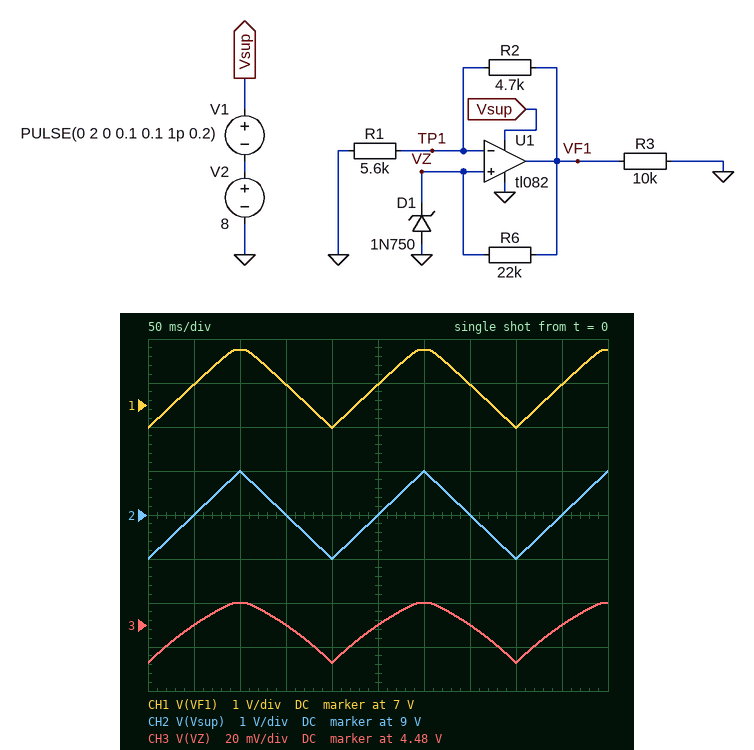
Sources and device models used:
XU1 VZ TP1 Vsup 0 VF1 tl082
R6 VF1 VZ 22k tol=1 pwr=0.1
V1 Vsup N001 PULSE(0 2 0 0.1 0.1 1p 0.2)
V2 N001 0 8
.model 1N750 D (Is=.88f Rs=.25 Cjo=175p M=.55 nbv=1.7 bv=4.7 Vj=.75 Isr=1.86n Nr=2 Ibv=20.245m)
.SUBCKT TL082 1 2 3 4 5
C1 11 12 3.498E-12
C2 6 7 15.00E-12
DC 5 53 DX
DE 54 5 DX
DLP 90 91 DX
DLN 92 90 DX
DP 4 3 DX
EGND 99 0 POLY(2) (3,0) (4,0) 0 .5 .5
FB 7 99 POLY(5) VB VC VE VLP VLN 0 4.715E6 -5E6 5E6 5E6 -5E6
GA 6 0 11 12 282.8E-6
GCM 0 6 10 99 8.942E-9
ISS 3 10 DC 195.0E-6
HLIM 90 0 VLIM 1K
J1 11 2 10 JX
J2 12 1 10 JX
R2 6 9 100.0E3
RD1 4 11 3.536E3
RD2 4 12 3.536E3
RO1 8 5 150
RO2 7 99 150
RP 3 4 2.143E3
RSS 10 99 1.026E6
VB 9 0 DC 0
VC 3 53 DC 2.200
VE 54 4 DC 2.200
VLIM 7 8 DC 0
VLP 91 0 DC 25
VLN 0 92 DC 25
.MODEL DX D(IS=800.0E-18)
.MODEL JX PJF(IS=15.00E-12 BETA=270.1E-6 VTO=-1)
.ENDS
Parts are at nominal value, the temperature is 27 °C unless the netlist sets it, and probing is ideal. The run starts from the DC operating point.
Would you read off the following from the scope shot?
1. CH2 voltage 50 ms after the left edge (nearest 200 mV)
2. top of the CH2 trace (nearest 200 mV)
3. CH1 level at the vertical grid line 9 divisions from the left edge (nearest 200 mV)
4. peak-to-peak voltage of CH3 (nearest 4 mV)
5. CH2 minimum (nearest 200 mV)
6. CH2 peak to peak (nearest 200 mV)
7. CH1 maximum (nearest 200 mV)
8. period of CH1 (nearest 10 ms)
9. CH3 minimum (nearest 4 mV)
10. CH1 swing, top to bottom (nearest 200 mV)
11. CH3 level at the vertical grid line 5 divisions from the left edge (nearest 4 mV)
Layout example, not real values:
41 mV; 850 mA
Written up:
9.0 V; 10.0 V; 7.4 V; 28 mV; 8.0 V; 2.0 V; 8.2 V; 200 ms; 4.464 V; 1.8 V; 4.480 V
